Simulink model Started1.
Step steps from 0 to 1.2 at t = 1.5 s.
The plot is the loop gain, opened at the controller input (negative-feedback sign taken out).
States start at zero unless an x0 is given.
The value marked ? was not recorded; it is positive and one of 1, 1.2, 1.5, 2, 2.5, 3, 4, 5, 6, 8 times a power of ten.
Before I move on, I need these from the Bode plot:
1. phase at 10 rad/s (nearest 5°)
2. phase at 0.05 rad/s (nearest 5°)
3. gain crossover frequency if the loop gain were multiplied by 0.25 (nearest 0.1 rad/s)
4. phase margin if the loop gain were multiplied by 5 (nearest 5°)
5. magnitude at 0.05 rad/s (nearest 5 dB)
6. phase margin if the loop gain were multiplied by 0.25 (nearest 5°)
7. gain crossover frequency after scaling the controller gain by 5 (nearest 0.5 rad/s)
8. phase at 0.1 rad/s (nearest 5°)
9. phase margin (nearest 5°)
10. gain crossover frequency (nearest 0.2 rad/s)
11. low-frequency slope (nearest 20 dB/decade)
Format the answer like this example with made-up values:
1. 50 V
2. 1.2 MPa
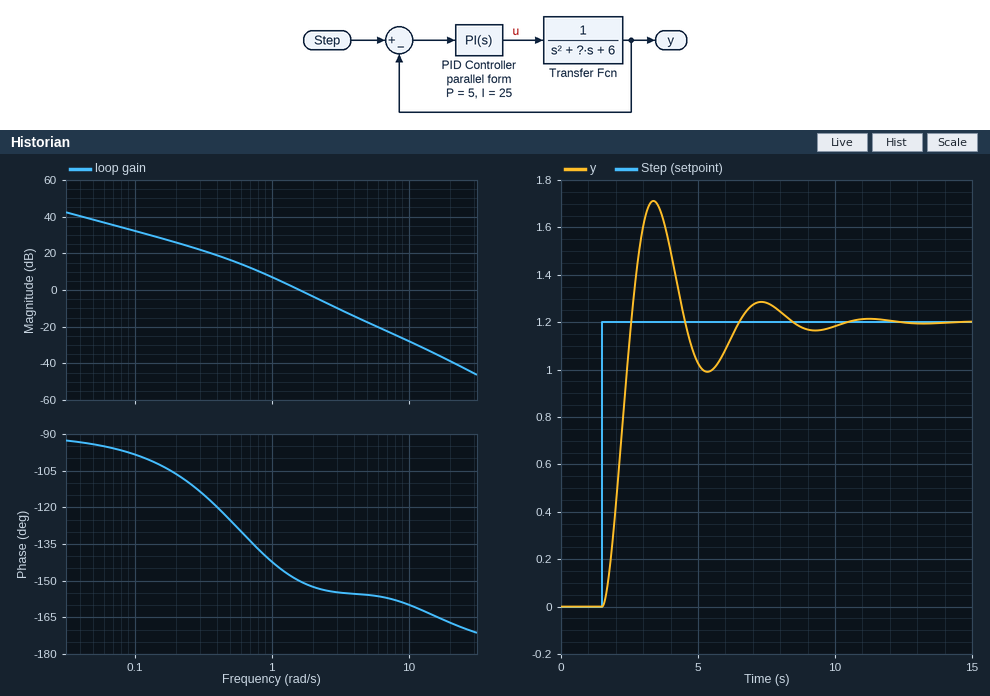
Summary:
1. -160°
2. -95°
3. 0.7 rad/s
4. 25°
5. 40 dB
6. 45°
7. 4.0 rad/s
8. -100°
9. 30°
10. 1.6 rad/s
11. -20 dB/decade
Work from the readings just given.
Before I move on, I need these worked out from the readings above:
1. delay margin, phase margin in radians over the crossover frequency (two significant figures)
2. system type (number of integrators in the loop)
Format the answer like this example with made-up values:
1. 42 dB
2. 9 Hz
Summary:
1. 0.33 s
2. 1
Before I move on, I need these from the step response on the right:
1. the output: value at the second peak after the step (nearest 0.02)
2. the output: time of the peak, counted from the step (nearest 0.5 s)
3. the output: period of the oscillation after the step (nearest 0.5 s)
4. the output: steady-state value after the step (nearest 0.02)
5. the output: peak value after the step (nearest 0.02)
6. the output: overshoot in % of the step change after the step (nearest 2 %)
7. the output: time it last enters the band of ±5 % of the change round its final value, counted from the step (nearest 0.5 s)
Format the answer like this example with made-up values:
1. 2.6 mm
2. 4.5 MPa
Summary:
1. 1.28
2. 2.0 s
3. 4.0 s
4. 1.20
5. 1.72
6. 42 %
7. 6.5 s
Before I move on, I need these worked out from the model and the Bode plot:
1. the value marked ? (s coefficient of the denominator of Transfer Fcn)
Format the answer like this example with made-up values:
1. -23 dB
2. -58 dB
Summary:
1. 10
